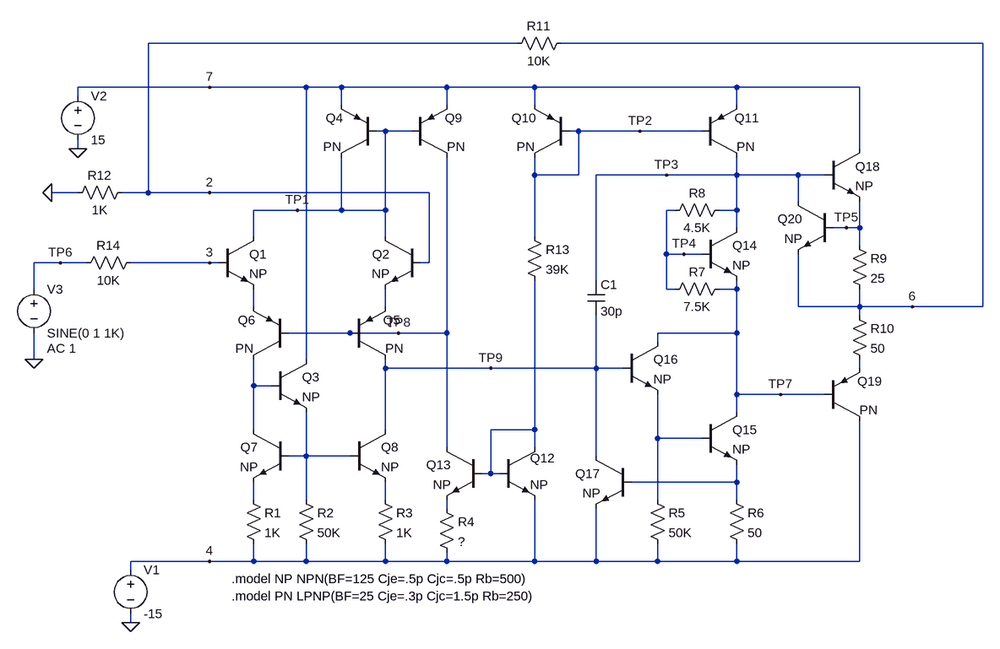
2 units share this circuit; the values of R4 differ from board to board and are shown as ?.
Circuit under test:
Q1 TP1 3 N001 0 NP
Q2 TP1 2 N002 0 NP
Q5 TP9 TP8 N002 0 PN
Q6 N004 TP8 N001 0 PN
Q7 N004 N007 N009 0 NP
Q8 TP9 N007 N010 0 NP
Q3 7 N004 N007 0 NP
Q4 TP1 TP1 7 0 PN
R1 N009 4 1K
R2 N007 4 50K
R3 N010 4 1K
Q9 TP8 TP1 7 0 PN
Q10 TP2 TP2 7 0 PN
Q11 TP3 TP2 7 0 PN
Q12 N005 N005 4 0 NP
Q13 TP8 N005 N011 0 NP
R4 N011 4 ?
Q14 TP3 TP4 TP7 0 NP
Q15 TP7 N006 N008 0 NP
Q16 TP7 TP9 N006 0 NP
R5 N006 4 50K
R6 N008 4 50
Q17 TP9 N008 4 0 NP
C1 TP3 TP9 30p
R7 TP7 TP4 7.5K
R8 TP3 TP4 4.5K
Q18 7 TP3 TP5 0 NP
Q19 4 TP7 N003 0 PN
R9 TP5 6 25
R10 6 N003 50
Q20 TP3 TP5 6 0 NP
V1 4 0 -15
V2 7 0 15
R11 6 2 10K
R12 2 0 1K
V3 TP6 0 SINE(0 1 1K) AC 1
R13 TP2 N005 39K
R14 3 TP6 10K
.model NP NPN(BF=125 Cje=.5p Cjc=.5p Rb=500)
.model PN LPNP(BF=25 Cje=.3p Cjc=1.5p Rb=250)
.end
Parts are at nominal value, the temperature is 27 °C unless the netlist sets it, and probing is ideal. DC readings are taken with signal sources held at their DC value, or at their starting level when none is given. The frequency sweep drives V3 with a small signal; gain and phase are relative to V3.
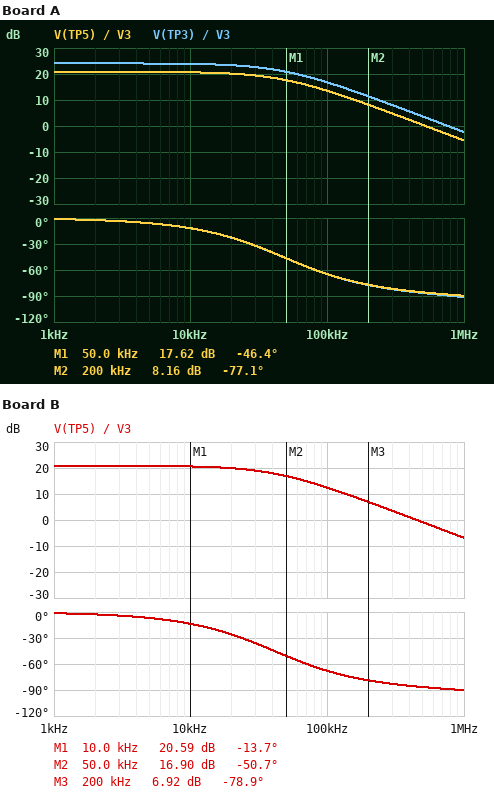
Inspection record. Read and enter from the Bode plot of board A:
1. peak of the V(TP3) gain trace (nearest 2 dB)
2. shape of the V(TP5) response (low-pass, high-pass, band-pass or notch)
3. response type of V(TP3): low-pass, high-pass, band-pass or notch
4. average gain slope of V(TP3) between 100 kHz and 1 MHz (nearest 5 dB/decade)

24 dB
low-pass
low-pass
-20 dB/decade
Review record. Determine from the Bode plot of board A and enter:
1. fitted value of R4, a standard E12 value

6.8 kΩ
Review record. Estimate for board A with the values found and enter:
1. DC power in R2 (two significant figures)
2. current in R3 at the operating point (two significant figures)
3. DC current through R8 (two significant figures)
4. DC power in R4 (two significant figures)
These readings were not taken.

8.6 µW
7.5 µA
110 µA
1.6 µW
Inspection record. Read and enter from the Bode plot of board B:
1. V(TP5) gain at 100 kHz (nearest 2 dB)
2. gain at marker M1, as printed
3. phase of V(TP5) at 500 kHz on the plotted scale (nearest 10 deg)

12 dB
20.59 dB
-90 deg
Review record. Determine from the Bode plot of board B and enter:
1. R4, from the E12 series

8.2 kΩ
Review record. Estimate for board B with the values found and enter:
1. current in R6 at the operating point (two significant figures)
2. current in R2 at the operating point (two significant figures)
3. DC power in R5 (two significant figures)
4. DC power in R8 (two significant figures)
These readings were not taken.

660 µA
13 µA
13 µW
51 µW
